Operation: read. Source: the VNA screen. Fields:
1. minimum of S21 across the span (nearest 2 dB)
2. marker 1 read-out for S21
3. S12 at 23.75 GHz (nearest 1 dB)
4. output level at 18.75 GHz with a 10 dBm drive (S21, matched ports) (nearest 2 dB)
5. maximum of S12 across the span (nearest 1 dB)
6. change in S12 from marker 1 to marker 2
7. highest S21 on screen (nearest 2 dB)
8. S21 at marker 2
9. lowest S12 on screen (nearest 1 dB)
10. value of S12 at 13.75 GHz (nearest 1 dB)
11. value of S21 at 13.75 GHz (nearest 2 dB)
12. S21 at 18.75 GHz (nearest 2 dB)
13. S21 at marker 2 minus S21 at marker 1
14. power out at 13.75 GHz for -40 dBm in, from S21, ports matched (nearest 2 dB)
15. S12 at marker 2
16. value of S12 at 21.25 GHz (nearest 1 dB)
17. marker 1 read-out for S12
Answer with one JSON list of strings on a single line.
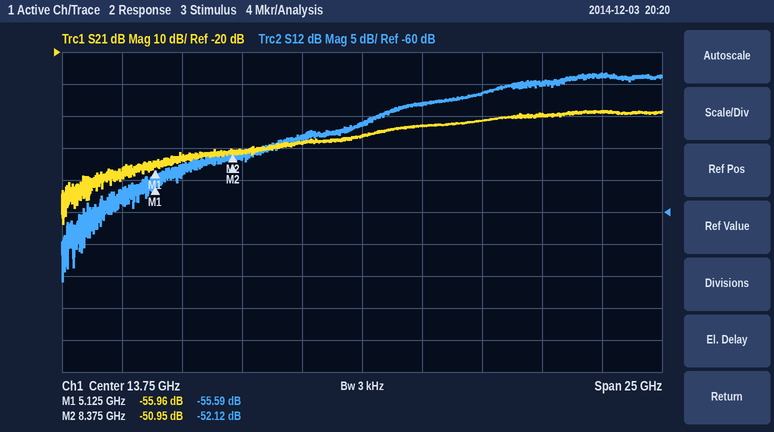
["-74 dB", "-55.96 dB", "-39 dB", "-32 dBm", "-38 dB", "3.47 dB", "-38 dB", "-50.95 dB", "-71 dB", "-46 dB", "-46 dB", "-42 dB", "5.01 dB", "-86 dBm", "-52.12 dB", "-40 dB", "-55.59 dB"]
